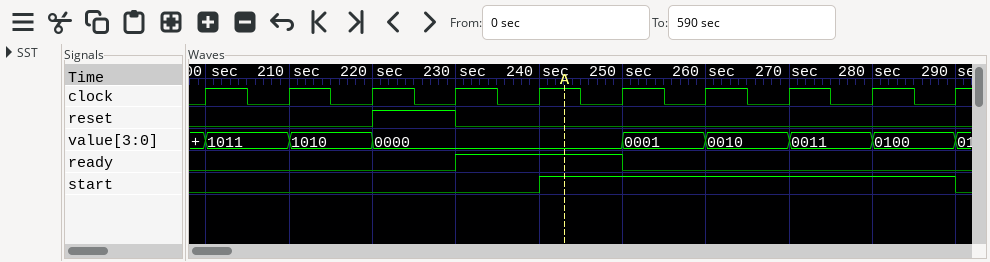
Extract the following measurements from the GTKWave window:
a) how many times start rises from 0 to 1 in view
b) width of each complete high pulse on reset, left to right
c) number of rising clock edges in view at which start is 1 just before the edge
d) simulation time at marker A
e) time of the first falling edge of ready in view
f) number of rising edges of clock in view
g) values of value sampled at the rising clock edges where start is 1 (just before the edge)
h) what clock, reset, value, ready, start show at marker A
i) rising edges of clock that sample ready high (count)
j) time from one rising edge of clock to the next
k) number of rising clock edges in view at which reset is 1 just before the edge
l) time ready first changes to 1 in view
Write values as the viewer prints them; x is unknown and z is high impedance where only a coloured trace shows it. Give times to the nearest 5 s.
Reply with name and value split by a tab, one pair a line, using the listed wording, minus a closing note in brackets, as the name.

how many times start rises from 0 to 1 in view	1
width of each complete high pulse on reset, left to right	10 s
number of rising clock edges in view at which start is 1 just before the edge	5
simulation time at marker A	245 s
time of the first falling edge of ready in view	250 s
number of rising edges of clock in view	10
values of value sampled at the rising clock edges where start is 1	0000, 0001, 0010, 0011, 0100
what clock, reset, value, ready, start show at marker A	clock=1, reset=0, value=0000, ready=1, start=1
rising edges of clock that sample ready high	2
time from one rising edge of clock to the next	10 s
number of rising clock edges in view at which reset is 1 just before the edge	1
time ready first changes to 1 in view	230 s
